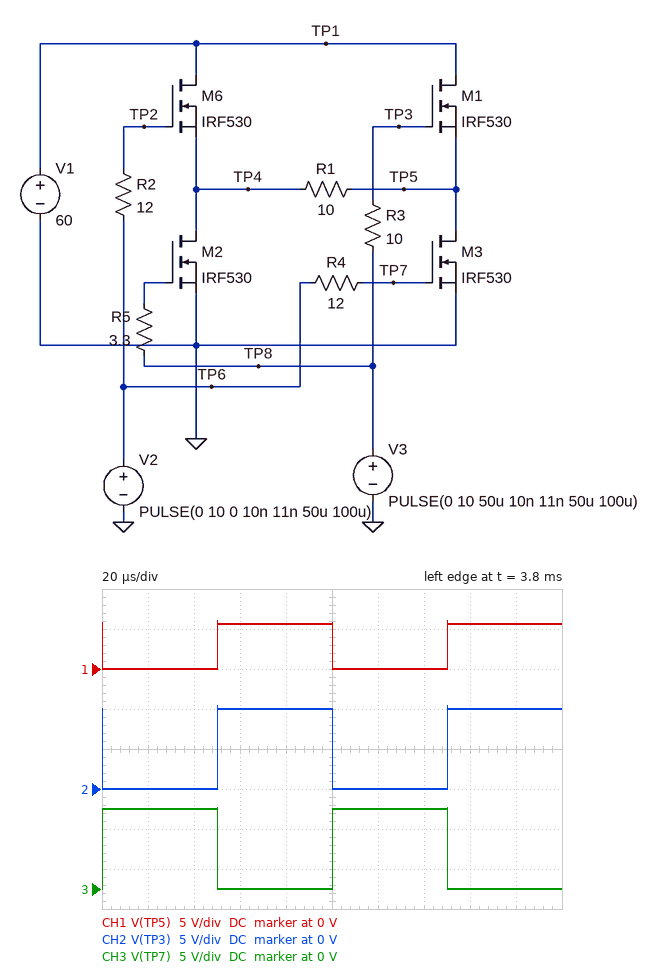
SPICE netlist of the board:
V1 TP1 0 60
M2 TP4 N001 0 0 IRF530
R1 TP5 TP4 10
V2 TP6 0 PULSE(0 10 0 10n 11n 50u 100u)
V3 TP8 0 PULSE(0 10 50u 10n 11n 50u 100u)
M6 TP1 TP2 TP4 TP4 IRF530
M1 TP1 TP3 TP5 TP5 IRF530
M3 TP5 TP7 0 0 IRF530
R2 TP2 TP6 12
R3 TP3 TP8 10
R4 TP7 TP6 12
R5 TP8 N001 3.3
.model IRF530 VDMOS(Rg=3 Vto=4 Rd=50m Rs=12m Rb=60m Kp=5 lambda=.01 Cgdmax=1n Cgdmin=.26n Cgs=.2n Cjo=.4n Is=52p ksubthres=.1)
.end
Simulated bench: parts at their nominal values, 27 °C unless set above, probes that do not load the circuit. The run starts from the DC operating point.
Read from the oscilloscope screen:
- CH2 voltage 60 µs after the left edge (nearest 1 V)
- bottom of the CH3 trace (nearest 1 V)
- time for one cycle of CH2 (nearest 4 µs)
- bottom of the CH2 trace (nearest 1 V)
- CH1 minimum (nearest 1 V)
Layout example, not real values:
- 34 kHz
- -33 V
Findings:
- 10 V
- 0 V
- 100 µs
- 0 V
- 0 V
